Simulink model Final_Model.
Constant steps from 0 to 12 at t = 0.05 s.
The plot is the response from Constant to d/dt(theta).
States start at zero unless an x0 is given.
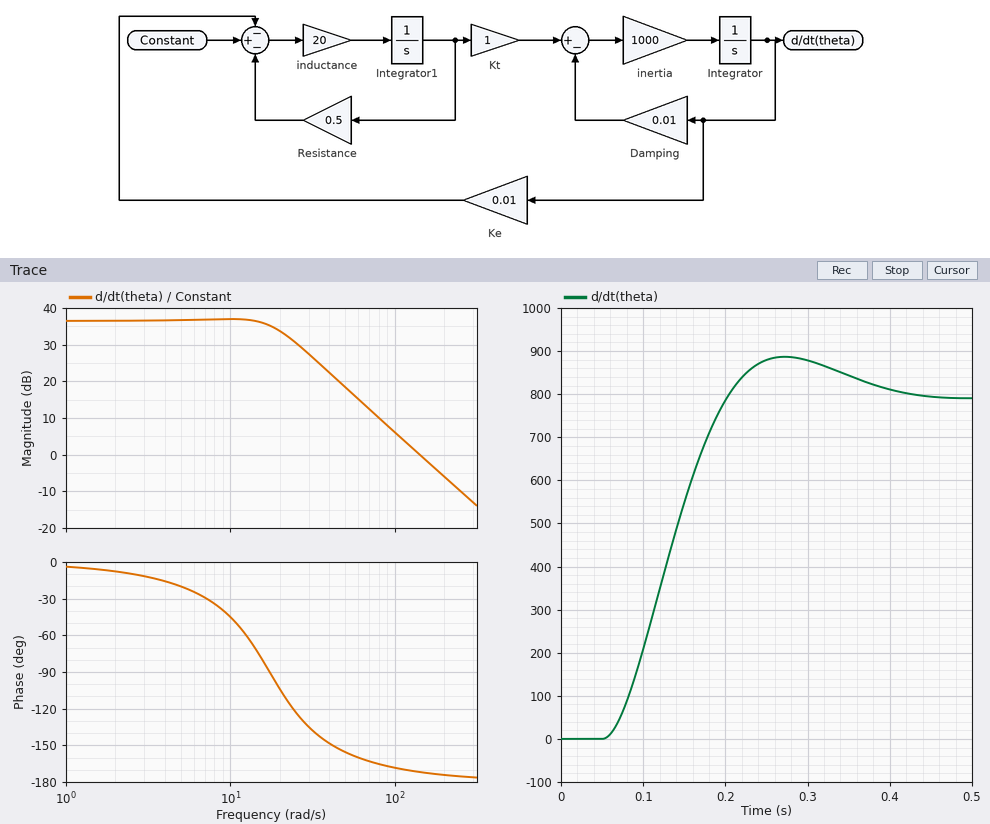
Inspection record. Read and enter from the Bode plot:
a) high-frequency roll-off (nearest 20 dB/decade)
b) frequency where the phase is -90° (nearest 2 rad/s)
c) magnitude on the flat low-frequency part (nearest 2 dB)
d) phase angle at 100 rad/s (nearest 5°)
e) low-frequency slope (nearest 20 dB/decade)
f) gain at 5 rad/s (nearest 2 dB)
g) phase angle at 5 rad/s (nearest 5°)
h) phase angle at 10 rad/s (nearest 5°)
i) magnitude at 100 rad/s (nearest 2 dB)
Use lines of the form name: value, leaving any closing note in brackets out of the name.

high-frequency roll-off: -40 dB/decade
frequency where the phase is -90°: 18 rad/s
magnitude on the flat low-frequency part: 36 dB
phase angle at 100 rad/s: -170°
low-frequency slope: 0 dB/decade
gain at 5 rad/s: 36 dB
phase angle at 5 rad/s: -20°
phase angle at 10 rad/s: -45°
magnitude at 100 rad/s: 6 dB
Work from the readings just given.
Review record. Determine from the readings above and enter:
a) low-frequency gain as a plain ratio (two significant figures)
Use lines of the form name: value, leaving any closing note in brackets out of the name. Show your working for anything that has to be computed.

low-frequency gain as a plain ratio: 10^(36 / 20) = 63
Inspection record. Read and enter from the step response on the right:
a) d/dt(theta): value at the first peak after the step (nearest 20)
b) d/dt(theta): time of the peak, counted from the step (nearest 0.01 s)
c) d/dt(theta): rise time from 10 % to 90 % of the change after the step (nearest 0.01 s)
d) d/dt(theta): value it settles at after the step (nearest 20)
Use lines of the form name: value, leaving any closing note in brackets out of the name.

d/dt(theta): value at the first peak after the step: 880
d/dt(theta): time of the peak, counted from the step: 0.22 s
d/dt(theta): rise time from 10 % to 90 % of the change after the step: 0.10 s
d/dt(theta): value it settles at after the step: 800
